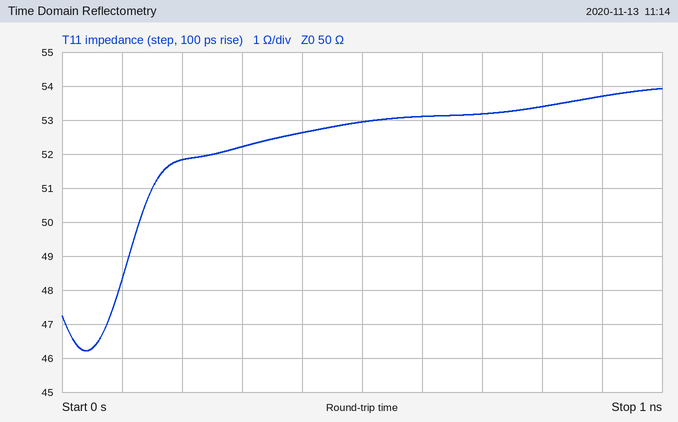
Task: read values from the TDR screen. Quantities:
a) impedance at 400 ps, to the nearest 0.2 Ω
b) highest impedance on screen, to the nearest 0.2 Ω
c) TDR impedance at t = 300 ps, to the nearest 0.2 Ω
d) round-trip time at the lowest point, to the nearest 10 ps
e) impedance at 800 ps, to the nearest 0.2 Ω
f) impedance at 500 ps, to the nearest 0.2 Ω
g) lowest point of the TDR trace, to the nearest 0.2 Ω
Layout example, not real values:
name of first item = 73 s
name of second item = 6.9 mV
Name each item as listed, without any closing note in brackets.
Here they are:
impedance at 400 ps, to the nearest 0.2 Ω = 52.6 Ω
highest impedance on screen, to the nearest 0.2 Ω = 54.0 Ω
TDR impedance at t = 300 ps, to the nearest 0.2 Ω = 52.2 Ω
round-trip time at the lowest point, to the nearest 10 ps = 40 ps
impedance at 800 ps, to the nearest 0.2 Ω = 53.4 Ω
impedance at 500 ps, to the nearest 0.2 Ω = 53.0 Ω
lowest point of the TDR trace, to the nearest 0.2 Ω = 46.2 Ω
